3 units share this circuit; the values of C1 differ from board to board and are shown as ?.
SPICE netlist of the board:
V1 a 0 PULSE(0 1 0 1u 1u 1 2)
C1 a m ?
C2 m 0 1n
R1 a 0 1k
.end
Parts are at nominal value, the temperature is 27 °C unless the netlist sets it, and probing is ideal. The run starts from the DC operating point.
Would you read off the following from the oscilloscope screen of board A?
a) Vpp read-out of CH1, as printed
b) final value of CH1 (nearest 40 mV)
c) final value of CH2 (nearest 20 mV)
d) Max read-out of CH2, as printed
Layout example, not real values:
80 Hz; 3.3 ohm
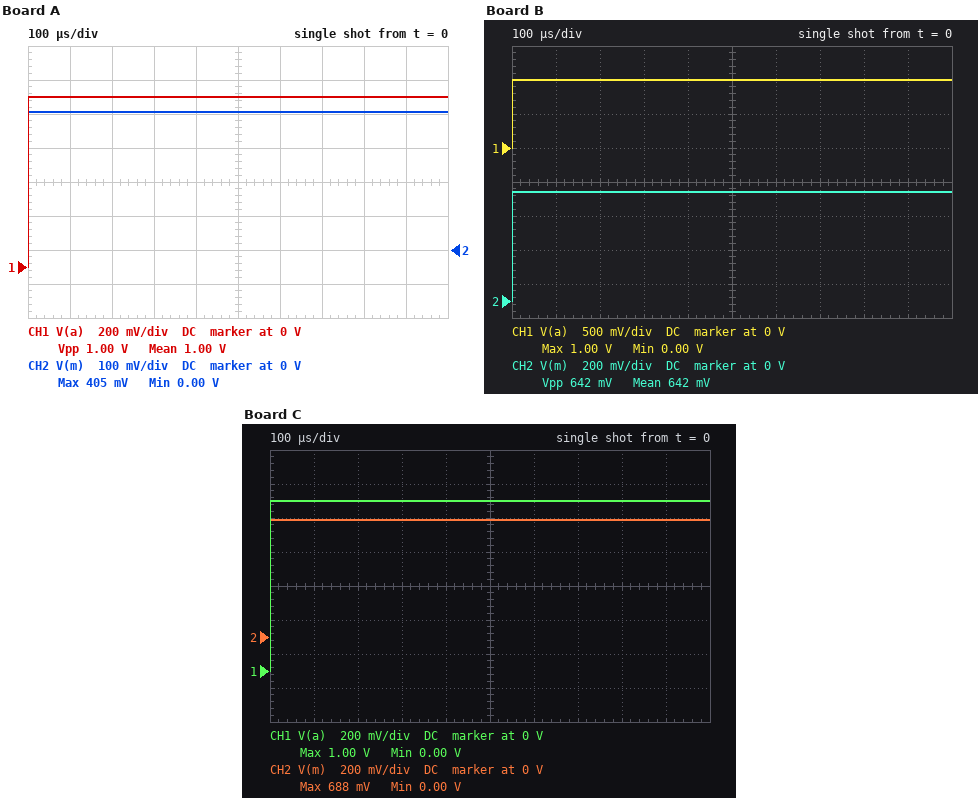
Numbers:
1.00 V; 1.00 V; 400 mV; 405 mV
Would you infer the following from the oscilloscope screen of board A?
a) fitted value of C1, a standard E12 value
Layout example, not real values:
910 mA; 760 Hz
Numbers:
680 pF
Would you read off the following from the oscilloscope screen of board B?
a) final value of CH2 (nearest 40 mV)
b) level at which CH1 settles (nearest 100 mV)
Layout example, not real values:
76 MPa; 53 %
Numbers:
640 mV; 1.0 V
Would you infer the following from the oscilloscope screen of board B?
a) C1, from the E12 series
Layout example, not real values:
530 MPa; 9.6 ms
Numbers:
1.8 nF
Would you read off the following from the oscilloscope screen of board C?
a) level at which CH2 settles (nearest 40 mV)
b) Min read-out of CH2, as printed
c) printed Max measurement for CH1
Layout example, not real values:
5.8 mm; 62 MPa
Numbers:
680 mV; 0.00 V; 1.00 V
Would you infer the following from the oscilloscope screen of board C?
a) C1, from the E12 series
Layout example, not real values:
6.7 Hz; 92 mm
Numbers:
2.2 nF
